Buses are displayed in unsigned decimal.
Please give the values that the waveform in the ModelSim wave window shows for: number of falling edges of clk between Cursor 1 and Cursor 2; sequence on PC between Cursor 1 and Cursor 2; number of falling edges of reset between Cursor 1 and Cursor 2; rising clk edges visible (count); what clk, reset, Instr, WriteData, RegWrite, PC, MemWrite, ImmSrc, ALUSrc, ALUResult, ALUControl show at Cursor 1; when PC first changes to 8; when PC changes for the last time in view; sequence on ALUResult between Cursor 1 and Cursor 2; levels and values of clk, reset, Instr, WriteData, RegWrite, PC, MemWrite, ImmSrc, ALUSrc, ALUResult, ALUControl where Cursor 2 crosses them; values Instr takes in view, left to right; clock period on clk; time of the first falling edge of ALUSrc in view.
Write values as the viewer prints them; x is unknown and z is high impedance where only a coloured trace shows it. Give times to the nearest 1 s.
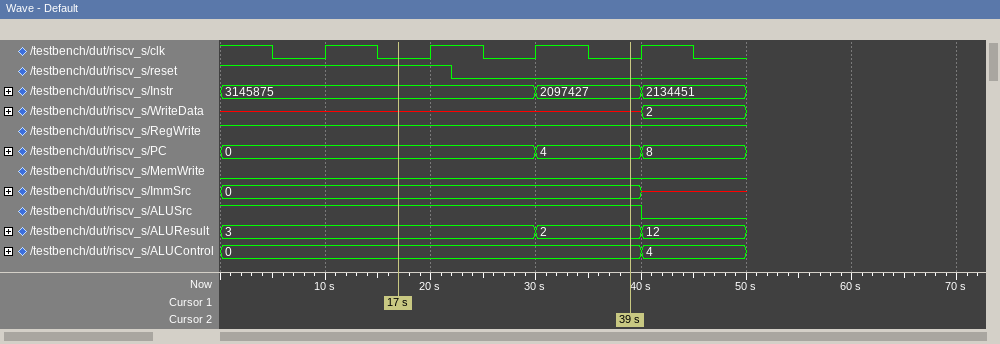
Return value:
2
0, 4
1
4
clk=0, reset=1, Instr=3145875, WriteData=x, RegWrite=1, PC=0, MemWrite=0, ImmSrc=0, ALUSrc=1, ALUResult=3, ALUControl=0
40 s
40 s
3, 2
clk=0, reset=0, Instr=2097427, WriteData=x, RegWrite=1, PC=4, MemWrite=0, ImmSrc=0, ALUSrc=1, ALUResult=2, ALUControl=0
3145875, 2097427, 2134451
10 s
40 s
